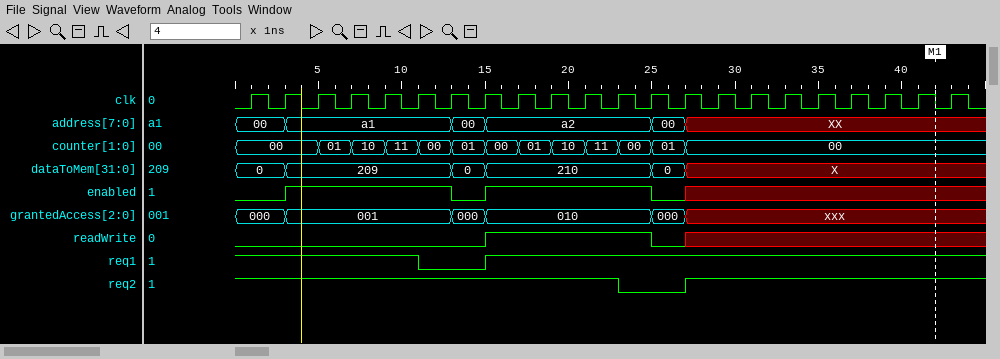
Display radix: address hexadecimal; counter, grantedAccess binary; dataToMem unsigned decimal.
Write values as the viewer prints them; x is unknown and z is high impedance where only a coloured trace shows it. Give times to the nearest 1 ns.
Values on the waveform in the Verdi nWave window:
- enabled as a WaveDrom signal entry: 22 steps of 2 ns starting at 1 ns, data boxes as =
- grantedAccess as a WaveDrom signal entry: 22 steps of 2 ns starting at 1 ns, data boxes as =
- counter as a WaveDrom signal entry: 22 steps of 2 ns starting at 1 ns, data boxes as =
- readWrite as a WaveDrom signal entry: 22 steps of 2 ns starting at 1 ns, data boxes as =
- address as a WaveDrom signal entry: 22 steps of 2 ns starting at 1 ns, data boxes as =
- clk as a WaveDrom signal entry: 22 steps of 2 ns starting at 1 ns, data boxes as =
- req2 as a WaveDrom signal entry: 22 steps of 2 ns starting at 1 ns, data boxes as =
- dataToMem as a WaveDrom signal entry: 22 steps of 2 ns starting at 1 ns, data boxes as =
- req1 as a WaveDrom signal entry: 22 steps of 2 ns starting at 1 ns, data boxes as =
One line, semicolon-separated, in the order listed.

{name: 'enabled', wave: '01....01....0x........'}; {name: 'grantedAccess', wave: '==....==....=x........', data: '000 001 000 010 000'}; {name: 'counter', wave: '=.============........', data: '00 01 10 11 00 01 00 01 10 11 00 01 00'}; {name: 'readWrite', wave: '0......1....0x........'}; {name: 'address', wave: '==....==....==........', data: '00 a1 00 a2 00 XX'}; {name: 'clk', wave: 'p.....................'}; {name: 'req2', wave: '1..........0.1........'}; {name: 'dataToMem', wave: '==....==....==........', data: '0 209 0 210 0 X'}; {name: 'req1', wave: '1....0.1..............'}
